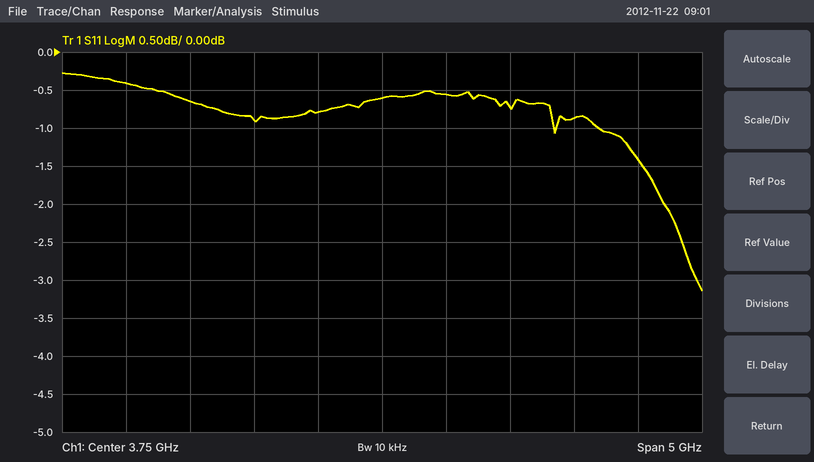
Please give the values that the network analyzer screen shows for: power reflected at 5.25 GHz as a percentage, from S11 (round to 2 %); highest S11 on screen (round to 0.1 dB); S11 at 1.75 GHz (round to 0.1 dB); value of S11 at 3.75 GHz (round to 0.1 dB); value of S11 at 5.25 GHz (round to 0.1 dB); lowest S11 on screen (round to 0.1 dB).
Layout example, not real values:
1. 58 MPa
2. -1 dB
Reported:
1. 82 %
2. -0.3 dB
3. -0.4 dB
4. -0.6 dB
5. -0.9 dB
6. -3.1 dB
